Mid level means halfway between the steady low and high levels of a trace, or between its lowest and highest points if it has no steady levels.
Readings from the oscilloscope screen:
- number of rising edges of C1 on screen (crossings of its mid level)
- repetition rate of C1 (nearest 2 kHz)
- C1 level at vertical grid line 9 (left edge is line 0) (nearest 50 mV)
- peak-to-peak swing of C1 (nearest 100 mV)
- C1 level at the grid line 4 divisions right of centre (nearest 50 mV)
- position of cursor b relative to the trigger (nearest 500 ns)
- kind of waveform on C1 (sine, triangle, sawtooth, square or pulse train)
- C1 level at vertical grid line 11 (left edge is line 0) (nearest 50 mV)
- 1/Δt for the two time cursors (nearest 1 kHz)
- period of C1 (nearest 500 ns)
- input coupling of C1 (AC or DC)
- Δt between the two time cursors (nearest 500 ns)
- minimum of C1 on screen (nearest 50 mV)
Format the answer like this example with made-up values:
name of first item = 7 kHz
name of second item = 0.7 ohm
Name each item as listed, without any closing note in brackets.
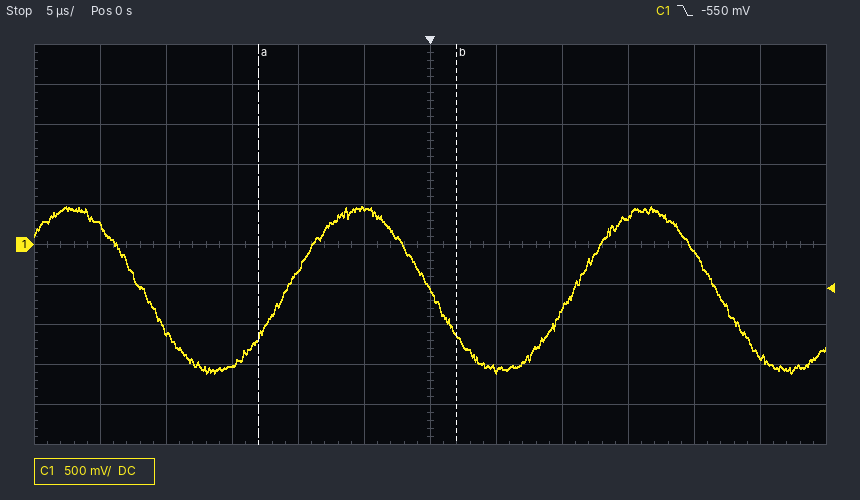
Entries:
number of rising edges of C1 on screen = 2
repetition rate of C1 = 46 kHz
C1 level at vertical grid line 9 (left edge is line 0) = 350 mV
peak-to-peak swing of C1 = 2.10 V
C1 level at the grid line 4 divisions right of centre = -100 mV
position of cursor b relative to the trigger = +2.0 µs
kind of waveform on C1 = sine
C1 level at vertical grid line 11 (left edge is line 0) = -1.40 V
1/Δt for the two time cursors = 67 kHz
period of C1 = 21.5 µs
input coupling of C1 = DC
Δt between the two time cursors = 15.0 µs
minimum of C1 on screen = -1.60 V
